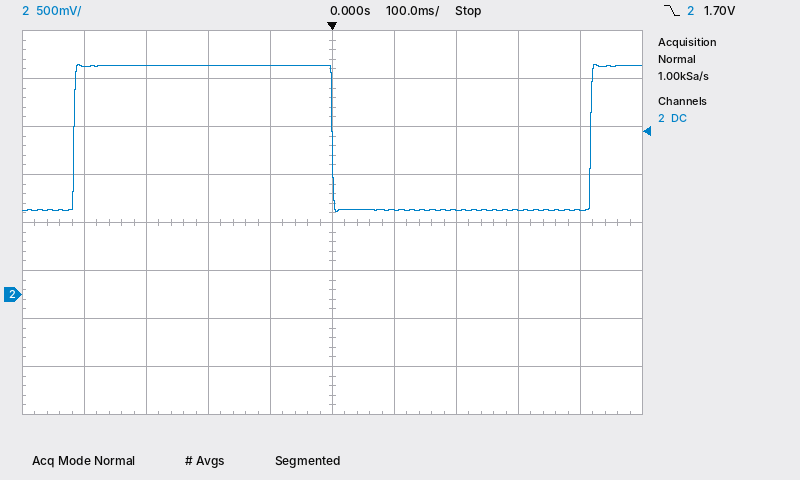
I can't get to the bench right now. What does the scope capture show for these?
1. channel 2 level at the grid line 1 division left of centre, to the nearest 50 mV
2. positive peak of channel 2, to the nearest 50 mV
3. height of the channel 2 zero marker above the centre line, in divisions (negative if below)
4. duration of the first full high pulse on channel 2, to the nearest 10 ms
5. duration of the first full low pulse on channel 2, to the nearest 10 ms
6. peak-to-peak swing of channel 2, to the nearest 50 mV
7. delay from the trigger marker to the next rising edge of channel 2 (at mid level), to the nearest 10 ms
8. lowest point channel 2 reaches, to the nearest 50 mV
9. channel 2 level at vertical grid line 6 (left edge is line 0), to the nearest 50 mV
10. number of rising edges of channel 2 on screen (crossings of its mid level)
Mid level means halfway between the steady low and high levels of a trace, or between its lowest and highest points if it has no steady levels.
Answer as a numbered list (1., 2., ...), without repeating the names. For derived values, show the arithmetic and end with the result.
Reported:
1. 2.40 V
2. 2.40 V
3. -1.5 div
4. 420 ms
5. 420 ms
6. 2.40 V − (850 mV) = 1.55 V
7. 420 ms
8. 850 mV
9. 900 mV
10. 2
